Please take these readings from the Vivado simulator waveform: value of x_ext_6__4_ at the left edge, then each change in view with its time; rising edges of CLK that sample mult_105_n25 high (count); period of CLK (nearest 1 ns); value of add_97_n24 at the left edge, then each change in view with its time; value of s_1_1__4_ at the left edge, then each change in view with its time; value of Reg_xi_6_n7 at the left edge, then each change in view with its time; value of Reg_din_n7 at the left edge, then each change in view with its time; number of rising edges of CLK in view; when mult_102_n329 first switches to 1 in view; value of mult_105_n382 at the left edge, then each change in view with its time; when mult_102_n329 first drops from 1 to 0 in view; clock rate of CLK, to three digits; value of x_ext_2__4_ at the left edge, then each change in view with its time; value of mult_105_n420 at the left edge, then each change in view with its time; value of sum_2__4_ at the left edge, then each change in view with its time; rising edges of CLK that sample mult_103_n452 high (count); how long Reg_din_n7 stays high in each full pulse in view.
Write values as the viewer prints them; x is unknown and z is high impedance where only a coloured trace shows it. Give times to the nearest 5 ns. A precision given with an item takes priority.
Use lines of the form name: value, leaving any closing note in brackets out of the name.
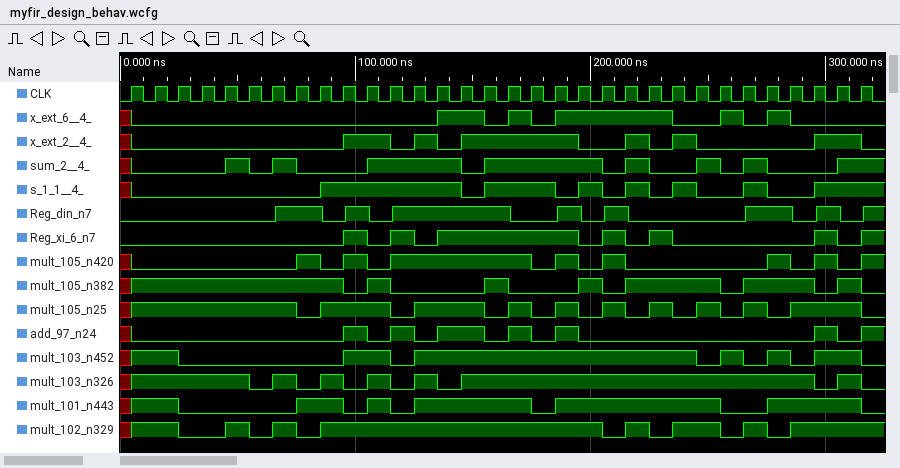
value of x_ext_6__4_ at the left edge, then each change in view with its time: x, 0 at 5 ns, 1 at 135 ns, 0 at 155 ns, 1 at 165 ns, 0 at 175 ns, 1 at 185 ns, 0 at 235 ns, 1 at 255 ns, 0 at 265 ns, 1 at 275 ns, 0 at 285 ns
rising edges of CLK that sample mult_105_n25 high: 22
period of CLK: 10 ns
value of add_97_n24 at the left edge, then each change in view with its time: x, 0 at 5 ns, 1 at 95 ns, 0 at 105 ns, 1 at 115 ns, 0 at 125 ns, 1 at 135 ns, 0 at 155 ns, 1 at 165 ns, 0 at 175 ns, 1 at 185 ns, 0 at 195 ns, 1 at 295 ns, 0 at 305 ns, 1 at 315 ns
value of s_1_1__4_ at the left edge, then each change in view with its time: x, 0 at 5 ns, 1 at 85 ns, 0 at 145 ns, 1 at 155 ns, 0 at 185 ns, 1 at 195 ns, 0 at 205 ns, 1 at 215 ns, 0 at 225 ns, 1 at 235 ns, 0 at 245 ns, 1 at 265 ns, 0 at 275 ns, 1 at 295 ns
value of Reg_xi_6_n7 at the left edge, then each change in view with its time: 0, 1 at 95 ns, 0 at 105 ns, 1 at 115 ns, 0 at 125 ns, 1 at 135 ns, 0 at 195 ns, 1 at 205 ns, 0 at 215 ns, 1 at 225 ns, 0 at 235 ns, 1 at 295 ns, 0 at 305 ns, 1 at 315 ns
value of Reg_din_n7 at the left edge, then each change in view with its time: 0, 1 at 65 ns, 0 at 85 ns, 1 at 95 ns, 0 at 105 ns, 1 at 115 ns, 0 at 165 ns, 1 at 185 ns, 0 at 195 ns, 1 at 205 ns, 0 at 215 ns, 1 at 265 ns, 0 at 285 ns, 1 at 295 ns, 0 at 305 ns, 1 at 315 ns
number of rising edges of CLK in view: 32
when mult_102_n329 first switches to 1 in view: 5 ns
value of mult_105_n382 at the left edge, then each change in view with its time: x, 1 at 5 ns, 0 at 95 ns, 1 at 105 ns, 0 at 115 ns, 1 at 155 ns, 0 at 165 ns, 1 at 195 ns, 0 at 205 ns, 1 at 215 ns, 0 at 255 ns, 1 at 265 ns, 0 at 295 ns, 1 at 305 ns, 0 at 315 ns
when mult_102_n329 first drops from 1 to 0 in view: 25 ns
clock rate of CLK, to three digits: 100 MHz
value of x_ext_2__4_ at the left edge, then each change in view with its time: x, 0 at 5 ns, 1 at 95 ns, 0 at 115 ns, 1 at 125 ns, 0 at 135 ns, 1 at 145 ns, 0 at 195 ns, 1 at 215 ns, 0 at 225 ns, 1 at 235 ns, 0 at 245 ns, 1 at 295 ns, 0 at 315 ns
value of mult_105_n420 at the left edge, then each change in view with its time: x, 0 at 5 ns, 1 at 75 ns, 0 at 85 ns, 1 at 95 ns, 0 at 105 ns, 1 at 115 ns, 0 at 175 ns, 1 at 185 ns, 0 at 195 ns, 1 at 205 ns, 0 at 215 ns, 1 at 275 ns, 0 at 285 ns, 1 at 295 ns, 0 at 305 ns, 1 at 315 ns
value of sum_2__4_ at the left edge, then each change in view with its time: x, 0 at 5 ns, 1 at 45 ns, 0 at 55 ns, 1 at 65 ns, 0 at 75 ns, 1 at 105 ns, 0 at 145 ns, 1 at 155 ns, 0 at 205 ns, 1 at 215 ns, 0 at 225 ns, 1 at 245 ns, 0 at 255 ns, 1 at 265 ns, 0 at 275 ns, 1 at 305 ns
rising edges of CLK that sample mult_103_n452 high: 20
how long Reg_din_n7 stays high in each full pulse in view: 20 ns, 10 ns, 50 ns, 10 ns, 10 ns, 20 ns, 10 ns
